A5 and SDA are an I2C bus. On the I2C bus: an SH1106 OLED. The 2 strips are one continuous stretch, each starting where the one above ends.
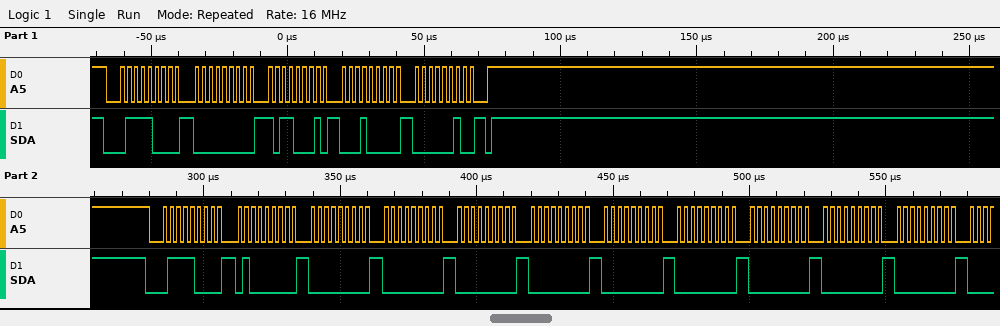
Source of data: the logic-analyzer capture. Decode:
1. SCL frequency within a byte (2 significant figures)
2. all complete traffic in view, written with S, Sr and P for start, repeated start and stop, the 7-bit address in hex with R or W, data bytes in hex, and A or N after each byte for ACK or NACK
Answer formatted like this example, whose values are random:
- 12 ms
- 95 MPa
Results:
- 400 kHz
- S 3CW A 00 A B1 A 10 A 02 A P S 3CW A 40 A 00 A 00 A 00 A 00 A 00 A 00 A 00 A 00 A 00 A
